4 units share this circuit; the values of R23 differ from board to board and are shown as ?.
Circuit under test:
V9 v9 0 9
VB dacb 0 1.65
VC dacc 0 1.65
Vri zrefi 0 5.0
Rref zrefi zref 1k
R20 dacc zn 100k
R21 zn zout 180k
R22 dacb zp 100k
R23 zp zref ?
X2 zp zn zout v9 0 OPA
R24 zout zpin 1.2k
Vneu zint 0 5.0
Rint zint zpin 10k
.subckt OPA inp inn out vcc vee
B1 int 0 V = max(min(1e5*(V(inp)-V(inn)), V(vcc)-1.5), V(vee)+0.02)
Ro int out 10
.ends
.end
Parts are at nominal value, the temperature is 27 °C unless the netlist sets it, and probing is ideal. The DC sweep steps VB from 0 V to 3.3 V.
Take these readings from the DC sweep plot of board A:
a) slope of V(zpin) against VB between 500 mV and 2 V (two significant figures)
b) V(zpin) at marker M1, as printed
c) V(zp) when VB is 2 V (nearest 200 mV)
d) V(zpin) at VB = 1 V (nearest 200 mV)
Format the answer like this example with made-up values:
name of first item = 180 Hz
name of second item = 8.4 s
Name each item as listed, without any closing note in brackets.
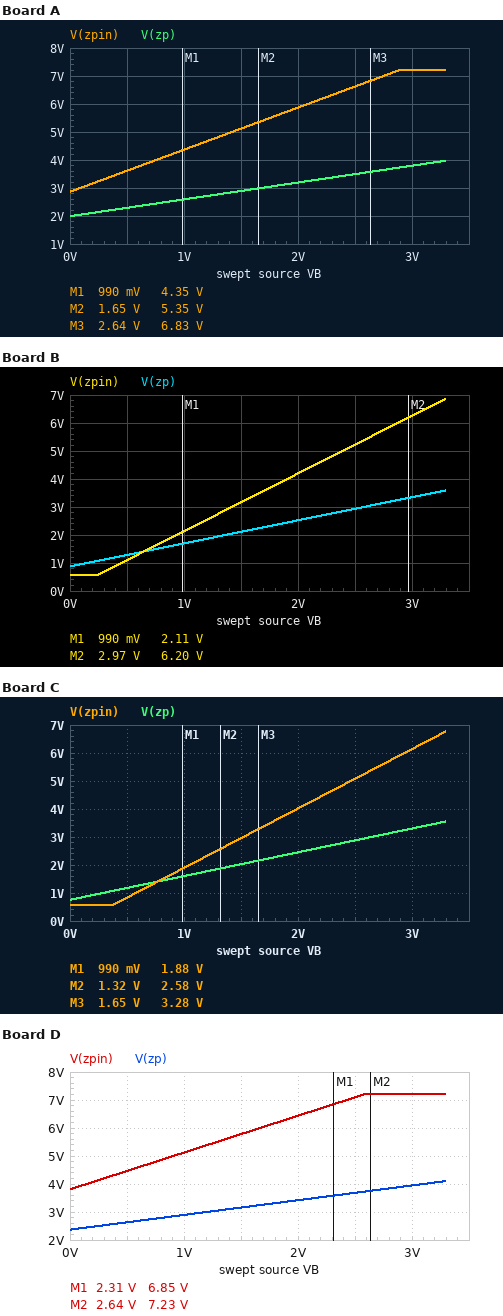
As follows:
slope of V(zpin) against VB between 500 mV and 2 V = 1.5 V/V
V(zpin) at marker M1, as printed = 4.35 V
V(zp) when VB is 2 V = 3.2 V
V(zpin) at VB = 1 V = 4.4 V
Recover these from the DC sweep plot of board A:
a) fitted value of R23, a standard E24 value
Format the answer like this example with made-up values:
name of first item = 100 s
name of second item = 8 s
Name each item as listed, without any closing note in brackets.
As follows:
fitted value of R23, a standard E24 value = 150 kΩ
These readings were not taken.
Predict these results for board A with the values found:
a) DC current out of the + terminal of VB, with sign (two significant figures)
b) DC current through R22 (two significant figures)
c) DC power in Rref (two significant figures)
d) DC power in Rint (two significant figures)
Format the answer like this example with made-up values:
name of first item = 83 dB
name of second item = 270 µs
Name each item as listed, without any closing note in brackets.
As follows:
DC current out of the + terminal of VB, with sign = -13 µA
DC current through R22 = 13 µA
DC power in Rref = 180 nW
DC power in Rint = 12 µW
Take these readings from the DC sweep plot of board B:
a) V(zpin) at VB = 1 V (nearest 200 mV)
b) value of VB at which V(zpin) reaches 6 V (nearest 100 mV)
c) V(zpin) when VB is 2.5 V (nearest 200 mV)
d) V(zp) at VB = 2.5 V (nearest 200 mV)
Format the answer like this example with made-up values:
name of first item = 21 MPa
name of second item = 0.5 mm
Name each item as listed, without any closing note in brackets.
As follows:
V(zpin) at VB = 1 V = 2.2 V
value of VB at which V(zpin) reaches 6 V = 2.9 V
V(zpin) when VB is 2.5 V = 5.2 V
V(zp) at VB = 2.5 V = 3.0 V
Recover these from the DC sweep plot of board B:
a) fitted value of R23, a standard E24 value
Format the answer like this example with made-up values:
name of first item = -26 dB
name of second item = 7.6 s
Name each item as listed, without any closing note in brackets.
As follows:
fitted value of R23, a standard E24 value = 470 kΩ
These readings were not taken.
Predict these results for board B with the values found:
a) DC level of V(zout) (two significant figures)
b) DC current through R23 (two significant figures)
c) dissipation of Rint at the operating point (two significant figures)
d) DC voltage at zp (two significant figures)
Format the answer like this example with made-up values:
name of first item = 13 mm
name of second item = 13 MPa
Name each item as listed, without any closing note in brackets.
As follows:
DC level of V(zout) = 3.3 V
DC current through R23 = 5.9 µA
dissipation of Rint at the operating point = 230 µW
DC voltage at zp = 2.2 V
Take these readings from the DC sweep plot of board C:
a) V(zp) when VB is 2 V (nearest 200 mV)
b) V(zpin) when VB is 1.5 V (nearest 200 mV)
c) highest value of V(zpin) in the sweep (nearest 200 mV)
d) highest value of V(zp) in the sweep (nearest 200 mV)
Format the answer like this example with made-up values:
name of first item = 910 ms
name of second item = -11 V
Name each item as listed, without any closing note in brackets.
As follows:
V(zp) when VB is 2 V = 2.4 V
V(zpin) when VB is 1.5 V = 3.0 V
highest value of V(zpin) in the sweep = 6.8 V
highest value of V(zp) in the sweep = 3.6 V
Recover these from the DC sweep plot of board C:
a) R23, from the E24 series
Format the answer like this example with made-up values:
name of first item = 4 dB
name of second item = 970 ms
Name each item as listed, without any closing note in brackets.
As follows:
R23, from the E24 series = 560 kΩ
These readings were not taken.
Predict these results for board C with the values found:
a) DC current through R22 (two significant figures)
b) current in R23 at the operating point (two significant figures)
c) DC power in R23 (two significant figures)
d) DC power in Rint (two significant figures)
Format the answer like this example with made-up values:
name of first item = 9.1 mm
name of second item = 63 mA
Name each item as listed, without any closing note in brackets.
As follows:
DC current through R22 = 5.1 µA
current in R23 at the operating point = 5.1 µA
DC power in R23 = 14 µW
DC power in Rint = 300 µW
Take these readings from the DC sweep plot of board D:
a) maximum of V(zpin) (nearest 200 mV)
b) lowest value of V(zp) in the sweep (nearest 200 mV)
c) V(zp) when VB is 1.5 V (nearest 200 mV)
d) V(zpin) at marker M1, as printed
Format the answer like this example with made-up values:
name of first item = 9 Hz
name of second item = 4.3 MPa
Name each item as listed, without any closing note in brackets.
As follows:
maximum of V(zpin) = 7.2 V
lowest value of V(zp) in the sweep = 2.4 V
V(zp) when VB is 1.5 V = 3.2 V
V(zpin) at marker M1, as printed = 6.85 V
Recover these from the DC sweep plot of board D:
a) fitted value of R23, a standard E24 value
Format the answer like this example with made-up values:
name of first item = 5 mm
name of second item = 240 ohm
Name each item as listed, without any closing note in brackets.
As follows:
fitted value of R23, a standard E24 value = 110 kΩ
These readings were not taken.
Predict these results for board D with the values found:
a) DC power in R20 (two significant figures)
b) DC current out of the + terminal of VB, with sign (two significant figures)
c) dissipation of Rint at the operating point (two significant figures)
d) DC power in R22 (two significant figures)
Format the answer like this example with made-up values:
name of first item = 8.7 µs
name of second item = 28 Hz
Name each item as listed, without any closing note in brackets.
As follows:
DC power in R20 = 25 µW
DC current out of the + terminal of VB, with sign = -16 µA
dissipation of Rint at the operating point = 96 µW
DC power in R22 = 25 µW
